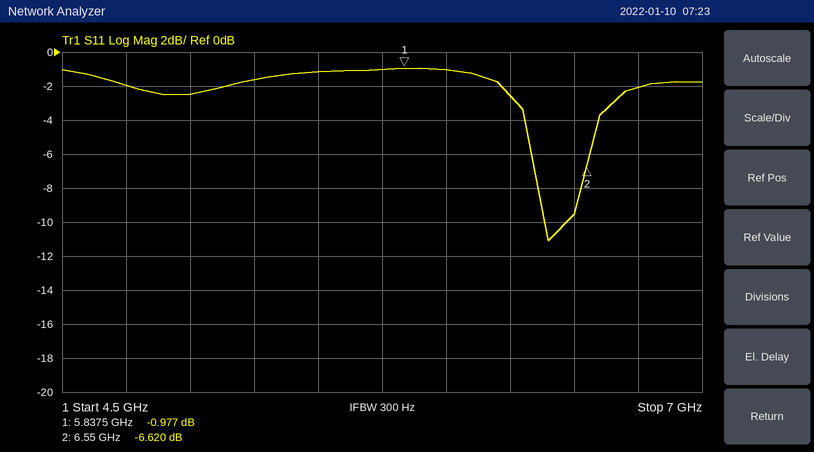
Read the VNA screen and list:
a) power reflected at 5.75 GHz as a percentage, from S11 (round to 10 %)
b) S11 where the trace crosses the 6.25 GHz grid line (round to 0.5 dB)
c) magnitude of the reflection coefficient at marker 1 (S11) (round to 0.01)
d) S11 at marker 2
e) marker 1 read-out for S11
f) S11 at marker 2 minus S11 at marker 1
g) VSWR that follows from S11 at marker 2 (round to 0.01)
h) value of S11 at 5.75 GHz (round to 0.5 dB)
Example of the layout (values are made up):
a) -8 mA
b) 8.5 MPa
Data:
a) 80 %
b) -2.5 dB
c) 0.89
d) -6.620 dB
e) -0.977 dB
f) -5.643 dB
g) 2.75
h) -1.0 dB
